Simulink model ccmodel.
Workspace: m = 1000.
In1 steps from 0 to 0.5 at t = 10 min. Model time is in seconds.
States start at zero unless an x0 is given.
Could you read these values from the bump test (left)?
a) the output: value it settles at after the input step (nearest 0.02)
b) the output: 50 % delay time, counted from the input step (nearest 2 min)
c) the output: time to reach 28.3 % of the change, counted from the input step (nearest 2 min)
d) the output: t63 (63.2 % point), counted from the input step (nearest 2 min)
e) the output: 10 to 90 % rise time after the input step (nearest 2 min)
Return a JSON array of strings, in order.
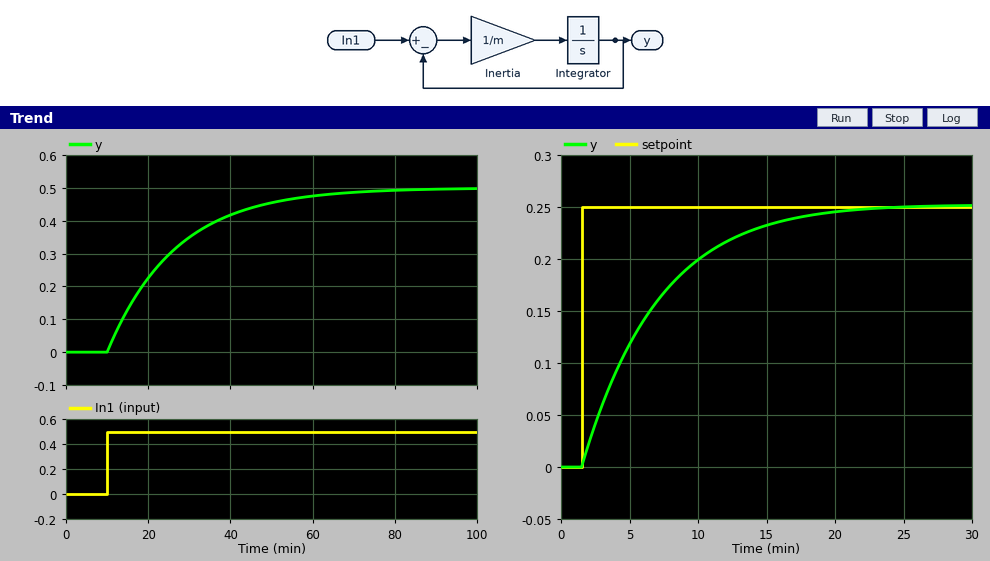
["0.50", "12 min", "6 min", "16 min", "36 min"]
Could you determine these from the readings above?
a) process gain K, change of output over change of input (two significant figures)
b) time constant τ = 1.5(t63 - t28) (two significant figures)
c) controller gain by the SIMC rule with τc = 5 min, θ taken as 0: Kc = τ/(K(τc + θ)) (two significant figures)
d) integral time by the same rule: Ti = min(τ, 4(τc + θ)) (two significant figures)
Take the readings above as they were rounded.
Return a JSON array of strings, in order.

["1.0", "15 min", "3.0", "15 min"]
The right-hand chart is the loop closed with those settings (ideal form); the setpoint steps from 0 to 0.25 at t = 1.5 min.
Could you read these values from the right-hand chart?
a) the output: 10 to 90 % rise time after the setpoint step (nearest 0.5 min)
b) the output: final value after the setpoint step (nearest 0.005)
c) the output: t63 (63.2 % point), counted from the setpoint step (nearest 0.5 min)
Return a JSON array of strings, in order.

["11.5 min", "0.250", "5.5 min"]
